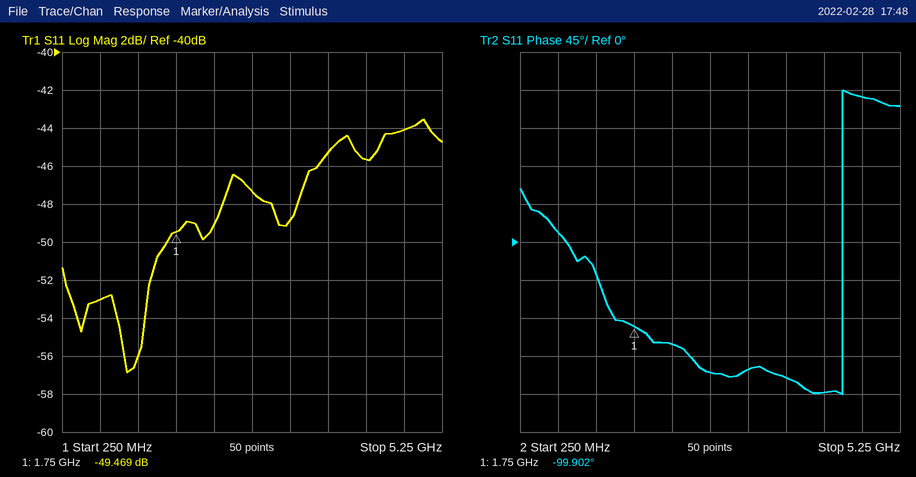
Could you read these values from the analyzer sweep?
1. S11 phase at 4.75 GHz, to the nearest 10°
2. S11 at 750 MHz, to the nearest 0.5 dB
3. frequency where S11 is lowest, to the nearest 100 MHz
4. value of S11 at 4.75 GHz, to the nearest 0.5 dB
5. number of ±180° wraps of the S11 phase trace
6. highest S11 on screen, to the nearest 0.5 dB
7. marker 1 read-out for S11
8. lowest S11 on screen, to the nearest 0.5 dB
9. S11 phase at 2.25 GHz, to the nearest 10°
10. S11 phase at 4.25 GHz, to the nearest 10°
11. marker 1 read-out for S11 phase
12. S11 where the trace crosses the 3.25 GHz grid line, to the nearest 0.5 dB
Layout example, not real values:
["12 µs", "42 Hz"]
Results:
["170°", "-53.0 dB", "1.1 GHz", "-44.0 dB", "1", "-43.5 dB", "-49.469 dB", "-57.0 dB", "-120°", "-180°", "-99.902°", "-49.0 dB"]
